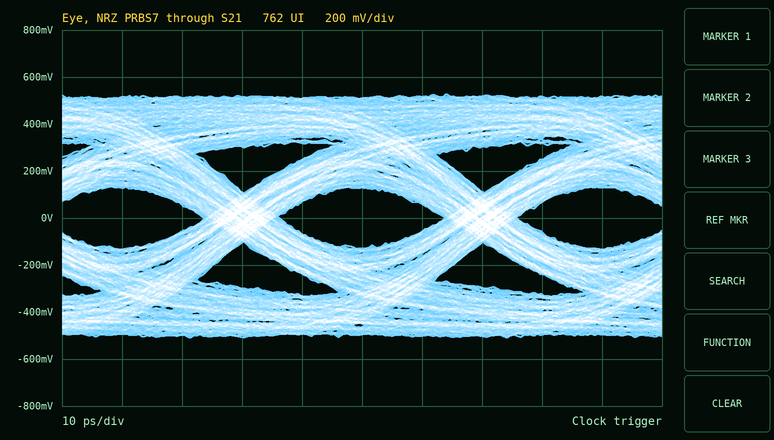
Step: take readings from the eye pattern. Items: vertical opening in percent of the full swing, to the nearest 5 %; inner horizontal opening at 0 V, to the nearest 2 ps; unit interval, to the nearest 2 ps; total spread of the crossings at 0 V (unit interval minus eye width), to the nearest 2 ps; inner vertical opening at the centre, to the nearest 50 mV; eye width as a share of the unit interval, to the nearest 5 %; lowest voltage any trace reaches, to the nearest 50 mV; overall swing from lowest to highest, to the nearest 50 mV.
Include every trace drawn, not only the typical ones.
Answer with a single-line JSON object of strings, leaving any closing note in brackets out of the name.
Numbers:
{"vertical opening in percent of the full swing, to the nearest 5 %": "25 %", "inner horizontal opening at 0 V, to the nearest 2 ps": "28 ps", "unit interval, to the nearest 2 ps": "40 ps", "total spread of the crossings at 0 V (unit interval minus eye width), to the nearest 2 ps": "12 ps", "inner vertical opening at the centre, to the nearest 50 mV": "250 mV", "eye width as a share of the unit interval, to the nearest 5 %": "70 %", "lowest voltage any trace reaches, to the nearest 50 mV": "-500 mV", "overall swing from lowest to highest, to the nearest 50 mV": "1.05 V"}
